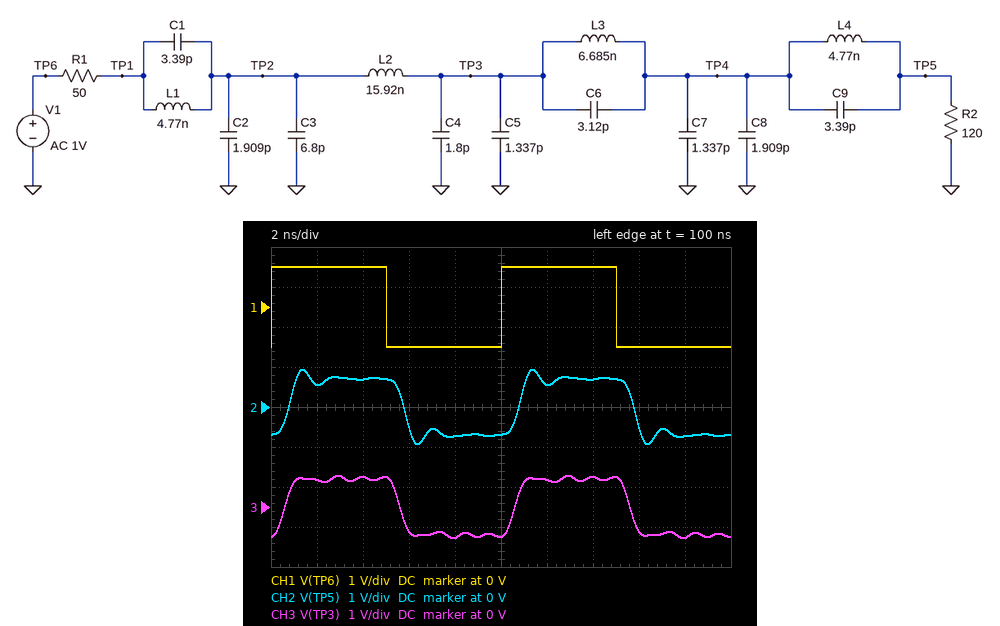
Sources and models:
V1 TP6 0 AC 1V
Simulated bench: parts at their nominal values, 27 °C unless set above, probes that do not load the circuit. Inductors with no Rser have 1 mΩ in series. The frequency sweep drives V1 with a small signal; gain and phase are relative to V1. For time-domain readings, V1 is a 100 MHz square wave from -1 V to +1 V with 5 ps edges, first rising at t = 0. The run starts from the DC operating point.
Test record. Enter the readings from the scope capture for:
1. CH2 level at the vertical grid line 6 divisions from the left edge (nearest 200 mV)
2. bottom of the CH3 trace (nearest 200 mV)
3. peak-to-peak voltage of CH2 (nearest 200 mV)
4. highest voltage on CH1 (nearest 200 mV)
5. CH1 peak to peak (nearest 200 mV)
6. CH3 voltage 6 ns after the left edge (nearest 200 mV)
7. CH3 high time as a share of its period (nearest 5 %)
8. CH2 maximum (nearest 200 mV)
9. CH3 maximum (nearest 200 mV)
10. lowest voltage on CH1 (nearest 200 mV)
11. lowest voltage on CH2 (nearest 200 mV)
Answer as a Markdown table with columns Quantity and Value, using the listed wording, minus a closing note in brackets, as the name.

| Quantity | Value |
|---|---|
| CH2 level at the vertical grid line 6 divisions from the left edge | 600 mV |
| bottom of the CH3 trace | -800 mV |
| peak-to-peak voltage of CH2 | 1.8 V |
| highest voltage on CH1 | 1.0 V |
| CH1 peak to peak | 2.0 V |
| CH3 voltage 6 ns after the left edge | -600 mV |
| CH3 high time as a share of its period | 50 % |
| CH2 maximum | 1.0 V |
| CH3 maximum | 800 mV |
| lowest voltage on CH1 | -1.0 V |
| lowest voltage on CH2 | -1.0 V |
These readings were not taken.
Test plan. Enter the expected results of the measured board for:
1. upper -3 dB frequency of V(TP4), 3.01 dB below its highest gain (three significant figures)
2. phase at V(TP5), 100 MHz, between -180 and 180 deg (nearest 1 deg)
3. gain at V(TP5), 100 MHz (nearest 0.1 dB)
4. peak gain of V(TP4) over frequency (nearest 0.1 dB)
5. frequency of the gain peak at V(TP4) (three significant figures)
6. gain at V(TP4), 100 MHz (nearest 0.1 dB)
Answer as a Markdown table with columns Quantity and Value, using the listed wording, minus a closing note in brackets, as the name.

| Quantity | Value |
|---|---|
| upper -3 dB frequency of V(TP4), 3.01 dB below its highest gain | 996 MHz |
| phase at V(TP5), 100 MHz, between -180 and 180 deg | -26 deg |
| gain at V(TP5), 100 MHz | -3.1 dB |
| peak gain of V(TP4) over frequency | -1.0 dB |
| frequency of the gain peak at V(TP4) | 986 MHz |
| gain at V(TP4), 100 MHz | -3.1 dB |
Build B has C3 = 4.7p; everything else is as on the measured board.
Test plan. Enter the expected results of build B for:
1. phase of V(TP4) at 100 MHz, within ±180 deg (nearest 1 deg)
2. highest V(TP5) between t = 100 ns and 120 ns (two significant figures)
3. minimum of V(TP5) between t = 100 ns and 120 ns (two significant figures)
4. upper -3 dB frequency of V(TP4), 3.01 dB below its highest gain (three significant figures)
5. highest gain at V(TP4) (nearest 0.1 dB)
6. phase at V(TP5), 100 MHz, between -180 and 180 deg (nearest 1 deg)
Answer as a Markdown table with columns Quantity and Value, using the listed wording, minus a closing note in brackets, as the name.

| Quantity | Value |
|---|---|
| phase of V(TP4) at 100 MHz, within ±180 deg | -22 deg |
| highest V(TP5) between t = 100 ns and 120 ns | 980 mV |
| minimum of V(TP5) between t = 100 ns and 120 ns | -980 mV |
| upper -3 dB frequency of V(TP4), 3.01 dB below its highest gain | 1.01 GHz |
| highest gain at V(TP4) | -0.9 dB |
| phase at V(TP5), 100 MHz, between -180 and 180 deg | -23 deg |
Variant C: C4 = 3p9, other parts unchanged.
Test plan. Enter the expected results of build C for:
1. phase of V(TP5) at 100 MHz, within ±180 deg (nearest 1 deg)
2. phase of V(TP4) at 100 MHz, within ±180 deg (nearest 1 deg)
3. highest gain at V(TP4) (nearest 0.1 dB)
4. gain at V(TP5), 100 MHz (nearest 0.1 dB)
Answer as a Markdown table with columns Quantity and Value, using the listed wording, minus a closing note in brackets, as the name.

| Quantity | Value |
|---|---|
| phase of V(TP5) at 100 MHz, within ±180 deg | -28 deg |
| phase of V(TP4) at 100 MHz, within ±180 deg | -27 deg |
| highest gain at V(TP4) | -2.2 dB |
| gain at V(TP5), 100 MHz | -3.2 dB |
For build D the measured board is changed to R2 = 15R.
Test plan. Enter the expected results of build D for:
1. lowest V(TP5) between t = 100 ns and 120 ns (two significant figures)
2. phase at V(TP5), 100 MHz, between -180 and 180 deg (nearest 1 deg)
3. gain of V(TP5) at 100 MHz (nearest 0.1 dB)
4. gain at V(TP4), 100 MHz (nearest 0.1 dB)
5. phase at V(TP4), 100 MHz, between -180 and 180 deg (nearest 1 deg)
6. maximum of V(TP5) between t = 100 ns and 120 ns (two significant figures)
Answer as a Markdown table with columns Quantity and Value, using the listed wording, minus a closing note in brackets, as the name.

| Quantity | Value |
|---|---|
| lowest V(TP5) between t = 100 ns and 120 ns | -300 mV |
| phase at V(TP5), 100 MHz, between -180 and 180 deg | -25 deg |
| gain of V(TP5) at 100 MHz | -12.6 dB |
| gain at V(TP4), 100 MHz | -12.4 dB |
| phase at V(TP4), 100 MHz, between -180 and 180 deg | -13 deg |
| maximum of V(TP5) between t = 100 ns and 120 ns | 300 mV |
